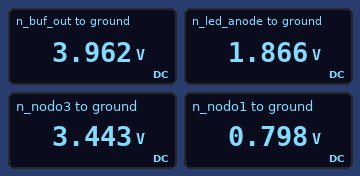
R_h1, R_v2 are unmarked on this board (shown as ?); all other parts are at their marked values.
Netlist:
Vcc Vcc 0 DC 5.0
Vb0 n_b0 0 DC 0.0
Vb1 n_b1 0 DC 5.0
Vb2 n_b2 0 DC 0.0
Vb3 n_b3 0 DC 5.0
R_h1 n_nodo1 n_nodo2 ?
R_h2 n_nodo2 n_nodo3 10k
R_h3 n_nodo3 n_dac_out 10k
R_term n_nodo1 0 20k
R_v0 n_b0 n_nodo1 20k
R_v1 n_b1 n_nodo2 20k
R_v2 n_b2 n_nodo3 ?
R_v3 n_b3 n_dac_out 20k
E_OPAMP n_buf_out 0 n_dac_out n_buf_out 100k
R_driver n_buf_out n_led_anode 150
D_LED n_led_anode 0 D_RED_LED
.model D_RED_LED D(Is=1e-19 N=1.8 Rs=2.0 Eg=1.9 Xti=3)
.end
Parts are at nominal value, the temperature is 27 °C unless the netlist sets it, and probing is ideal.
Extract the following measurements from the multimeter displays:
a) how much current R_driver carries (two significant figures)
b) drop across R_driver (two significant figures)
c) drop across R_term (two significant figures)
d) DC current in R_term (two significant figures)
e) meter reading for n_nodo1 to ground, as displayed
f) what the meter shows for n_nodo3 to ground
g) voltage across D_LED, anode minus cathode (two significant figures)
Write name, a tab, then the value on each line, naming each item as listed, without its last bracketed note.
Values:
how much current R_driver carries	14 mA
drop across R_driver	2.1 V
drop across R_term	800 mV
DC current in R_term	40 µA
meter reading for n_nodo1 to ground, as displayed	0.798 V
what the meter shows for n_nodo3 to ground	3.443 V
voltage across D_LED, anode minus cathode	1.9 V
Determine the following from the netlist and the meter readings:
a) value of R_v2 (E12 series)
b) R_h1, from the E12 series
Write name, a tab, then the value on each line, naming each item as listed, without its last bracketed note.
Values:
value of R_v2	68 kΩ
R_h1, from the E12 series	33 kΩ
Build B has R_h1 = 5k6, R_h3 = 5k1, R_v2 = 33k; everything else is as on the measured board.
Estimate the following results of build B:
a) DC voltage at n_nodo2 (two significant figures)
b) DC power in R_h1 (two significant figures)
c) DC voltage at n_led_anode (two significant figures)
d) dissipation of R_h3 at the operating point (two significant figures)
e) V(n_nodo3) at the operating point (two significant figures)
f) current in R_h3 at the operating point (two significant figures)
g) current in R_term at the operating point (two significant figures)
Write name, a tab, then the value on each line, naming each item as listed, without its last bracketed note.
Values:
DC voltage at n_nodo2	2.4 V
DC power in R_h1	130 µW
DC voltage at n_led_anode	1.8 V
dissipation of R_h3 at the operating point	48 µW
V(n_nodo3) at the operating point	2.6 V
current in R_h3 at the operating point	97 µA
current in R_term at the operating point	76 µA
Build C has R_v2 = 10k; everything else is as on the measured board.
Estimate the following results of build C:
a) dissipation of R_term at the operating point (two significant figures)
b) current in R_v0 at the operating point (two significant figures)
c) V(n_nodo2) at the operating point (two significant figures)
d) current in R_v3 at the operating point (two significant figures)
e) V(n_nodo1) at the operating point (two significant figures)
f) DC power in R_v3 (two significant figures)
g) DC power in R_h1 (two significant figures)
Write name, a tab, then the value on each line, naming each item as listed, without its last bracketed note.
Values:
dissipation of R_term at the operating point	16 µW
current in R_v0 at the operating point	29 µA
V(n_nodo2) at the operating point	2.5 V
current in R_v3 at the operating point	110 µA
V(n_nodo1) at the operating point	570 mV
DC power in R_v3	230 µW
DC power in R_h1	110 µW
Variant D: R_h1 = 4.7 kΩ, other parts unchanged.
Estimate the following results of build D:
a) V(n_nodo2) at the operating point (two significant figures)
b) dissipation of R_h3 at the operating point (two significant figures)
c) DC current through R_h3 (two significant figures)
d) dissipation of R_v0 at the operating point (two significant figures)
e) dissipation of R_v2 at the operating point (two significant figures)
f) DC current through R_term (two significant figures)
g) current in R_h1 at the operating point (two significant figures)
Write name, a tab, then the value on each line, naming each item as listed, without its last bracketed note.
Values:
V(n_nodo2) at the operating point	2.4 V
dissipation of R_h3 at the operating point	56 µW
DC current through R_h3	75 µA
dissipation of R_v0 at the operating point	130 µW
dissipation of R_v2 at the operating point	110 µW
DC current through R_term	82 µA
current in R_h1 at the operating point	160 µA
